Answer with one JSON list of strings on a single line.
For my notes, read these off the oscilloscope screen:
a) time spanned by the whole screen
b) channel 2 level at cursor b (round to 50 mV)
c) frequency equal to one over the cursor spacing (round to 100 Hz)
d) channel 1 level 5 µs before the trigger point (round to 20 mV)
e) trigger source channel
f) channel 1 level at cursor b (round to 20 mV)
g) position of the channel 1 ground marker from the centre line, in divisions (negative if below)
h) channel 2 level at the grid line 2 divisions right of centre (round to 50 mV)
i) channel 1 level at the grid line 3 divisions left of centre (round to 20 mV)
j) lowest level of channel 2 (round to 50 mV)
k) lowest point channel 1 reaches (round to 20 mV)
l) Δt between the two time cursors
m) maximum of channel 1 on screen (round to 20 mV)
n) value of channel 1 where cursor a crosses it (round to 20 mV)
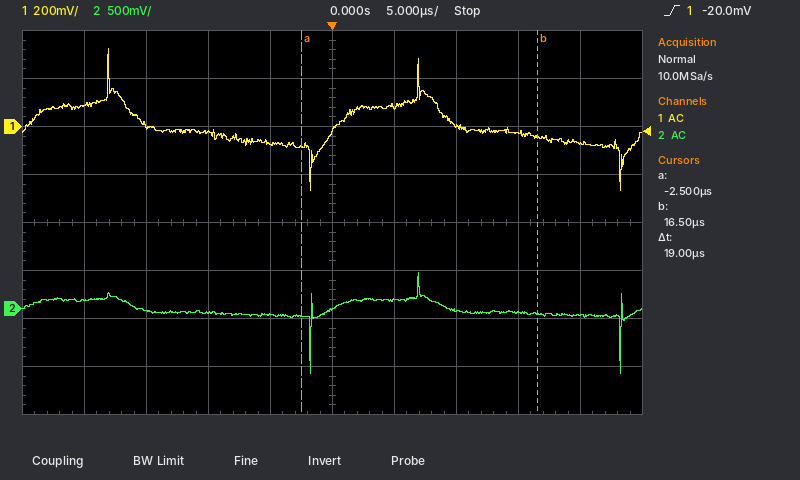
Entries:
["50 µs", "-50 mV", "52.6 kHz", "-80 mV", "channel 1", "-40 mV", "+2.0 div", "0 mV", "0 mV", "-650 mV", "-260 mV", "19 µs", "320 mV", "-80 mV"]
